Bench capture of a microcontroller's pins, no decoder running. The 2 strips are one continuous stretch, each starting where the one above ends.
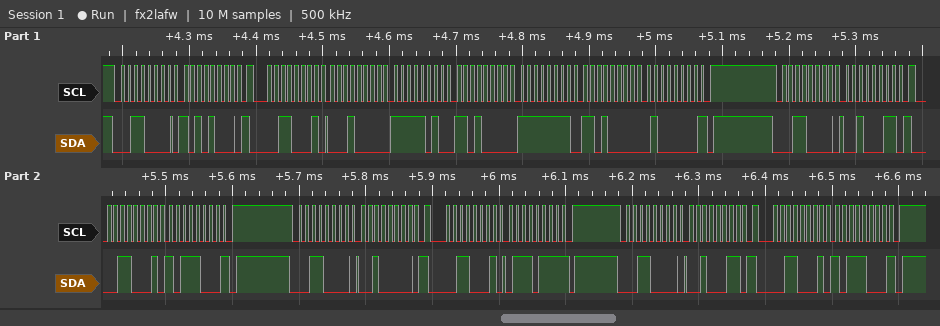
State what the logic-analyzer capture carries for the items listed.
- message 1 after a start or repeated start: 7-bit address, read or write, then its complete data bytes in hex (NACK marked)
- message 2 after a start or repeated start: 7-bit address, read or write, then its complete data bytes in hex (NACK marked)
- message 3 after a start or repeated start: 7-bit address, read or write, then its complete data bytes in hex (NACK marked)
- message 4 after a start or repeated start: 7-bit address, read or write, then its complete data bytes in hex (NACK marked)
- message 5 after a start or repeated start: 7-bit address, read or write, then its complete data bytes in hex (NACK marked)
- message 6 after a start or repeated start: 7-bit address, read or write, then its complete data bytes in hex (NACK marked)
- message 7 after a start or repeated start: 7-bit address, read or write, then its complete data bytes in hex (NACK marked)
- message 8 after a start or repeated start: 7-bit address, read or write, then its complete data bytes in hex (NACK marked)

0x18 write: A8
0x18 read: 10 FA D0 FF D0 40 NACK
0x18 write: 23
0x18 read: B8 NACK
0x18 write: 20
0x18 read: 77 NACK
0x18 write: 23
0x18 read: B8 NACK
